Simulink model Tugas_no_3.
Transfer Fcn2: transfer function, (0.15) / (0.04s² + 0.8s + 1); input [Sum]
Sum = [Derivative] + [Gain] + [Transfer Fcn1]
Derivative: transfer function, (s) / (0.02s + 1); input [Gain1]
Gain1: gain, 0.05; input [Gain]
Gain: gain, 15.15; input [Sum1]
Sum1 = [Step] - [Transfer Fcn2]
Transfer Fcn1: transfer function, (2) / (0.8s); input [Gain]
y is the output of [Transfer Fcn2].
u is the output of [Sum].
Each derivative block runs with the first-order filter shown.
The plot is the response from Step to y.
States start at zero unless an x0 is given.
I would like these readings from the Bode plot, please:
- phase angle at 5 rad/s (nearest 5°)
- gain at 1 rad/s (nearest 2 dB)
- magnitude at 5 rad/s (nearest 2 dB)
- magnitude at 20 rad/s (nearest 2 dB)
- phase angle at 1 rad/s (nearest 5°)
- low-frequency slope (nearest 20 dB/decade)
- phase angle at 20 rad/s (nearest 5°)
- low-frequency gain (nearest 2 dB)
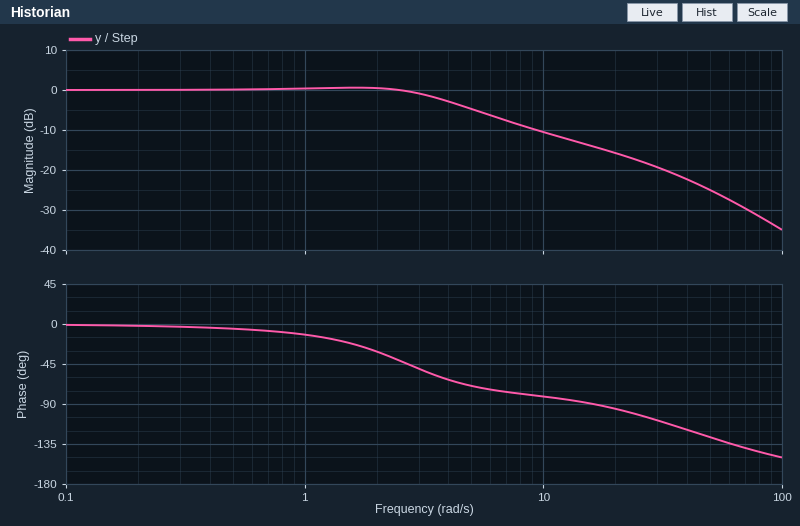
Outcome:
-70°
0 dB
-4 dB
-16 dB
-10°
0 dB/decade
-95°
0 dB
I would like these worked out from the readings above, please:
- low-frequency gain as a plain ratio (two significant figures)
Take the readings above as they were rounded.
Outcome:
1.0
